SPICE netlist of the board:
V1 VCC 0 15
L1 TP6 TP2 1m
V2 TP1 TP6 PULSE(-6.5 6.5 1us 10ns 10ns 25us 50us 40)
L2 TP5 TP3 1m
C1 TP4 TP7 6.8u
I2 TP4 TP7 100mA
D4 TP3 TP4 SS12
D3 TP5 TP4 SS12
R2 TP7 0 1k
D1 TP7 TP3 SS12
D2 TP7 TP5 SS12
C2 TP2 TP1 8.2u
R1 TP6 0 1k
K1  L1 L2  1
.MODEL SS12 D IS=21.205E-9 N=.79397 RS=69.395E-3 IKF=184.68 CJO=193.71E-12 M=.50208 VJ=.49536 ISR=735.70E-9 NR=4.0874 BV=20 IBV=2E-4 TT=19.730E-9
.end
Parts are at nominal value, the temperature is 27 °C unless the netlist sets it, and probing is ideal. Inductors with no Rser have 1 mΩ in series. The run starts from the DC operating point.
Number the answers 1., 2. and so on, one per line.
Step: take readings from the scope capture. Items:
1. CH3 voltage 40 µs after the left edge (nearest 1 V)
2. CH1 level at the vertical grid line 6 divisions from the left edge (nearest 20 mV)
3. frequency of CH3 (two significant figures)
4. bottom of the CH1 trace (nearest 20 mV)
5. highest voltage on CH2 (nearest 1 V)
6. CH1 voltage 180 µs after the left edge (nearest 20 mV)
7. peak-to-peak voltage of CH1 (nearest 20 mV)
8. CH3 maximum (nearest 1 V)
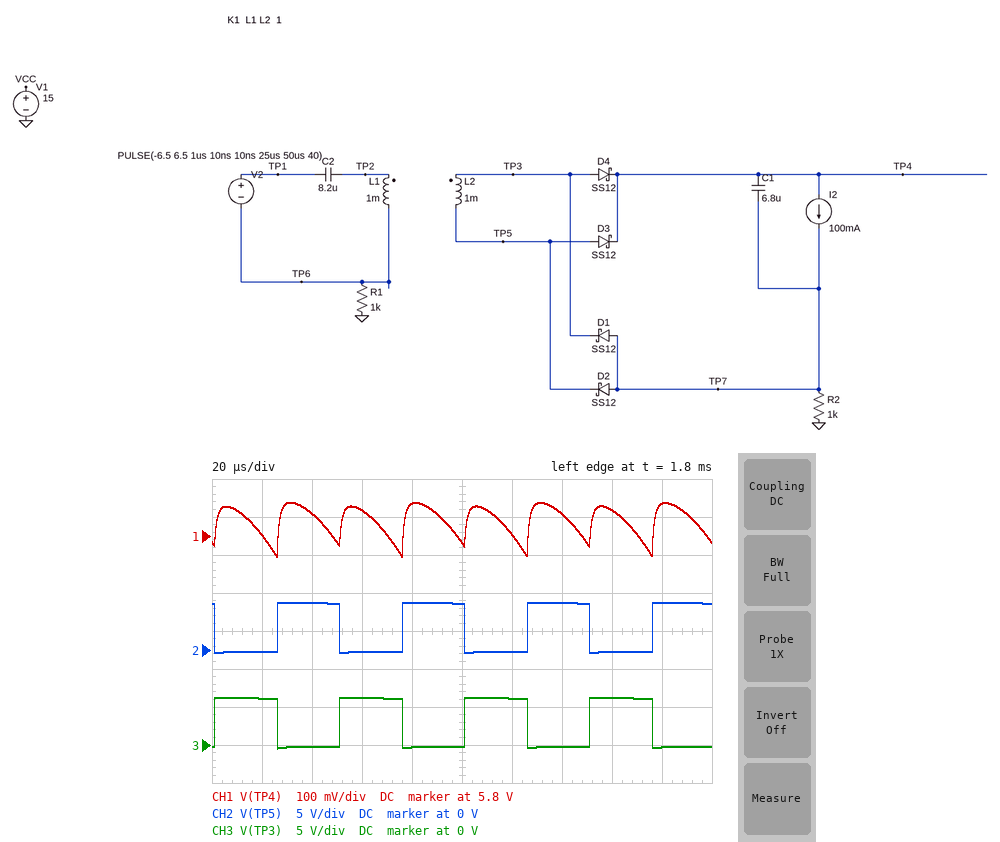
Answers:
1. 0 V
2. 5.80 V
3. 20 kHz
4. 5.74 V
5. 6 V
6. 5.88 V
7. 140 mV
8. 6 V
